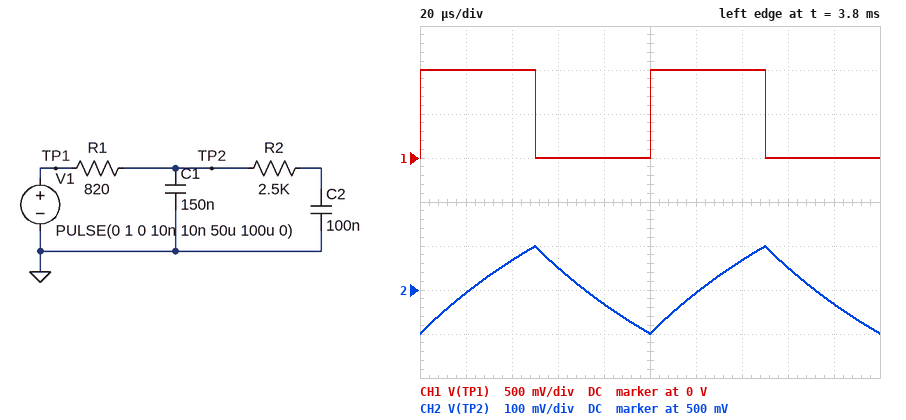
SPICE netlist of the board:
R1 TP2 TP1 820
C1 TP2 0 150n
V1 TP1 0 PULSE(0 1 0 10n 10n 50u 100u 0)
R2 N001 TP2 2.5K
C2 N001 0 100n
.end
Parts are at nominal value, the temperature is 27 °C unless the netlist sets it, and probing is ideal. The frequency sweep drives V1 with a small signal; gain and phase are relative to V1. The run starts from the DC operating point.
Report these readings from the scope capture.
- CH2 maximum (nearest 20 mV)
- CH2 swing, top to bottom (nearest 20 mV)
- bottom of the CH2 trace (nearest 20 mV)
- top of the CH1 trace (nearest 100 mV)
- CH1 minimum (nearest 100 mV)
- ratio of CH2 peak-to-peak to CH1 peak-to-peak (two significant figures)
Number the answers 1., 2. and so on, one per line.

1. 600 mV
2. 200 mV
3. 400 mV
4. 1.0 V
5. 0 V
6. 0.20
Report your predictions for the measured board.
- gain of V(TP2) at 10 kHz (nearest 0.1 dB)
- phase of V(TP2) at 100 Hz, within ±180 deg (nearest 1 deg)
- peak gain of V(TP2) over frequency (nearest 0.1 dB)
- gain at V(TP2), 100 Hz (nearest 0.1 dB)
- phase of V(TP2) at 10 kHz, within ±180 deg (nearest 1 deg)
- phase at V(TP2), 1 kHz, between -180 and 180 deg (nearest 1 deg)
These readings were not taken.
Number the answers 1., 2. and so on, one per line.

1. -17.9 dB
2. -7 deg
3. 0 dB
4. -0.1 dB
5. -80 deg
6. -37 deg
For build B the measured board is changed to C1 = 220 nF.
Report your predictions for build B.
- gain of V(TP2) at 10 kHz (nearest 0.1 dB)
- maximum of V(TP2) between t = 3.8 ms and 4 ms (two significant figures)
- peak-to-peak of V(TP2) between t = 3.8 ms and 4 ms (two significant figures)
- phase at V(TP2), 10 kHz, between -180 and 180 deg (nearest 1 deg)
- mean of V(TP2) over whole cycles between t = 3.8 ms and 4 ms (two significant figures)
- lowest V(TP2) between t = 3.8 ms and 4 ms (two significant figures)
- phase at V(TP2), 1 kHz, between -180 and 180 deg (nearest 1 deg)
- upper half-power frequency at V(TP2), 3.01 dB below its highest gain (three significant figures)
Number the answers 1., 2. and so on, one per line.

1. -21.2 dB
2. 570 mV
3. 140 mV
4. -83 deg
5. 500 mV
6. 430 mV
7. -46 deg
8. 583 Hz
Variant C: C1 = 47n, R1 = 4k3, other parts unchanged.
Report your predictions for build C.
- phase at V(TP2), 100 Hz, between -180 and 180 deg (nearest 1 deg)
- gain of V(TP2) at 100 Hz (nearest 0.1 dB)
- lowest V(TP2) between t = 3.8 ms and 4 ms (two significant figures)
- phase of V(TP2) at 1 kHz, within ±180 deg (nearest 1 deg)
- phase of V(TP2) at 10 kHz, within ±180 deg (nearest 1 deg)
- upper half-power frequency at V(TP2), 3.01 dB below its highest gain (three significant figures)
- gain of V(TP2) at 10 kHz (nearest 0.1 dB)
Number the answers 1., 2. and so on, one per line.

1. -21 deg
2. -0.9 dB
3. 440 mV
4. -43 deg
5. -78 deg
6. 213 Hz
7. -22.3 dB
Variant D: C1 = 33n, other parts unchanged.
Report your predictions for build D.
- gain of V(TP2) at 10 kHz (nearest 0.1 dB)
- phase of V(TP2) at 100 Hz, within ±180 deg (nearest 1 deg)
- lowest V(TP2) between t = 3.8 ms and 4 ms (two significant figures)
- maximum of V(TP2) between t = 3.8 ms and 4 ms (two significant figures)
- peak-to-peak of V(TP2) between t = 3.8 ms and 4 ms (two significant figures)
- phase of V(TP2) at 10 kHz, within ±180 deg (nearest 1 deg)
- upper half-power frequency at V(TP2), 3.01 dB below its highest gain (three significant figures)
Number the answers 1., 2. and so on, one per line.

1. -6.7 dB
2. -4 deg
3. 180 mV
4. 820 mV
5. 630 mV
6. -52 deg
7. 2.69 kHz
